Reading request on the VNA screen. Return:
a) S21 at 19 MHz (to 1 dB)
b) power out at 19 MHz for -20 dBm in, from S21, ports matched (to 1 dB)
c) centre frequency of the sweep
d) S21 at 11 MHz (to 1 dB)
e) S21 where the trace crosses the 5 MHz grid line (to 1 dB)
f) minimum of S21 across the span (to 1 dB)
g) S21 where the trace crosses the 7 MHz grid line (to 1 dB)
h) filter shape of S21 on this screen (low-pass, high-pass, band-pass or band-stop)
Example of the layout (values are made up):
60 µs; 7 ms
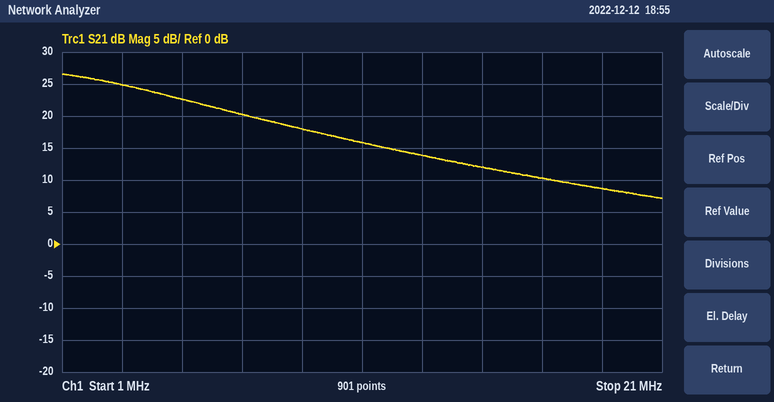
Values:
9 dB; -11 dBm; 11 MHz; 16 dB; 23 dB; 7 dB; 20 dB; low-pass
